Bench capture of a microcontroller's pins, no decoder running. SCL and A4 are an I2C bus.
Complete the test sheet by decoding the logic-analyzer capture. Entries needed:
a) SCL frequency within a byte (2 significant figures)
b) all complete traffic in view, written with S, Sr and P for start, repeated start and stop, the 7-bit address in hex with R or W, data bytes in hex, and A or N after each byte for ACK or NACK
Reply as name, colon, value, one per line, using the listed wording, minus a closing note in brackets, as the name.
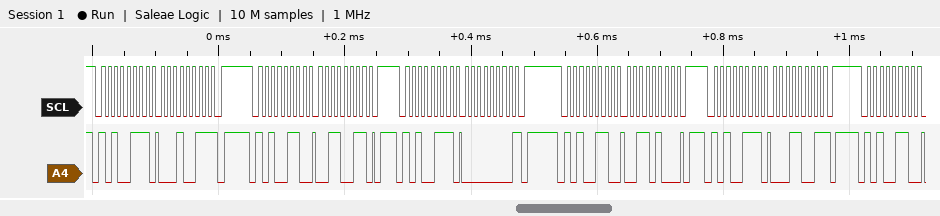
SCL frequency within a byte: 100 kHz
all complete traffic in view, written with S, Sr and P for start, repeated start and stop, the 7-bit address in hex with R or W, data bytes in hex, and A or N after each byte for ACK or NACK: S 53R A 13 N P S 53W A 33 A P S 53R A 00 N P S 53W A 34 A P S 53R A 19 N P S 53W A
